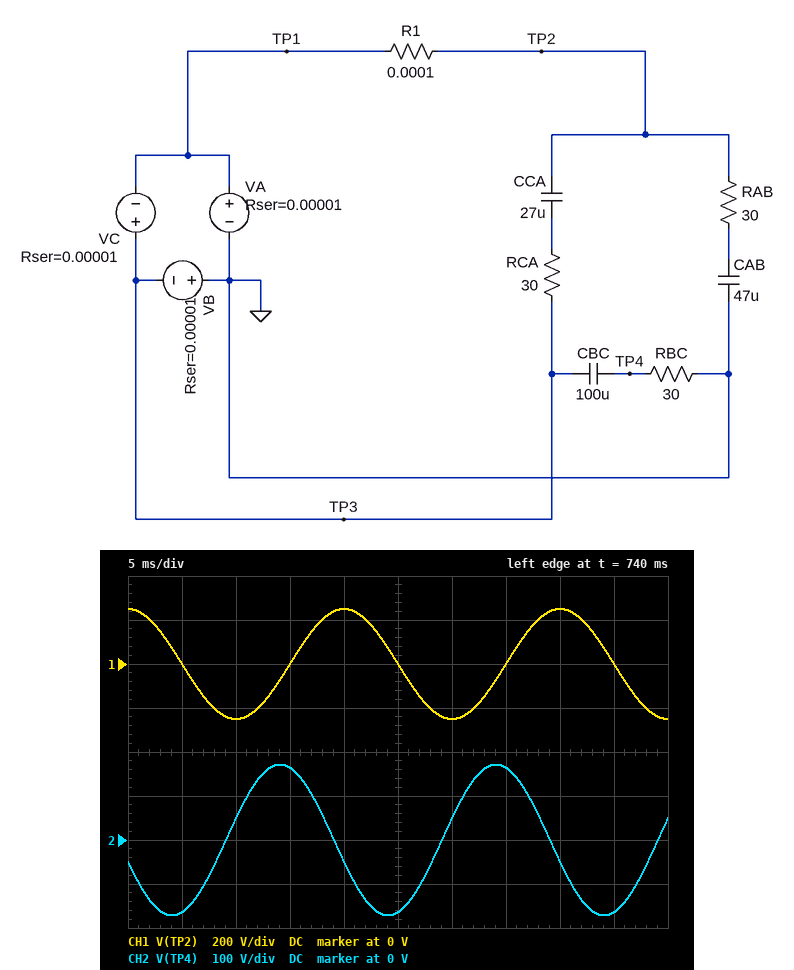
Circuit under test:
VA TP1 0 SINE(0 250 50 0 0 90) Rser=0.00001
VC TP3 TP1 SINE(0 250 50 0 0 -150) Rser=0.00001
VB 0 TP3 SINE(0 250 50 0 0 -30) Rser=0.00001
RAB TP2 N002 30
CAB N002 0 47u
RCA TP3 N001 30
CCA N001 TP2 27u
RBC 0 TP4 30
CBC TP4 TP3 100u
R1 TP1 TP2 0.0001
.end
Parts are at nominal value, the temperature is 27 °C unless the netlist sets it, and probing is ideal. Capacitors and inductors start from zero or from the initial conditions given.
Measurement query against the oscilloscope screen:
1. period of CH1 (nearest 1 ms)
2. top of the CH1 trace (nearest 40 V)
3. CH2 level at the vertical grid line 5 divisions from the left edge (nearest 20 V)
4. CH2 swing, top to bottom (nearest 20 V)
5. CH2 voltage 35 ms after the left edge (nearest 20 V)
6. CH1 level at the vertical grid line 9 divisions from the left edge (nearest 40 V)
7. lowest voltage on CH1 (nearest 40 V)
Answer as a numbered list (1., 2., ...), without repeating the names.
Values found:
1. 20 ms
2. 240 V
3. -160 V
4. 340 V
5. 160 V
6. 0 V
7. -240 V
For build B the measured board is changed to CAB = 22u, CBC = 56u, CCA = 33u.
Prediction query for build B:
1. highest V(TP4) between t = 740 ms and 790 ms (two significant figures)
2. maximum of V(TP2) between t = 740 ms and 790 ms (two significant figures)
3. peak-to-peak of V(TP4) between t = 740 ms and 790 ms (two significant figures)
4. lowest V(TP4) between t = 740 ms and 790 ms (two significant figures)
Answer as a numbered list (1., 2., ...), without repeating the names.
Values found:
1. 120 V
2. 250 V
3. 230 V
4. -120 V
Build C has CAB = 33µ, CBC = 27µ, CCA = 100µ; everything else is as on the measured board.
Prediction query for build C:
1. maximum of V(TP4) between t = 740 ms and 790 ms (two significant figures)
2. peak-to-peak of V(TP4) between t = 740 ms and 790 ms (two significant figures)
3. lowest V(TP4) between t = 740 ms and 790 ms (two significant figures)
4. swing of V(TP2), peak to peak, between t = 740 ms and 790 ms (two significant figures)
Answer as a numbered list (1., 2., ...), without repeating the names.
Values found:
1. 62 V
2. 120 V
3. -62 V
4. 500 V
